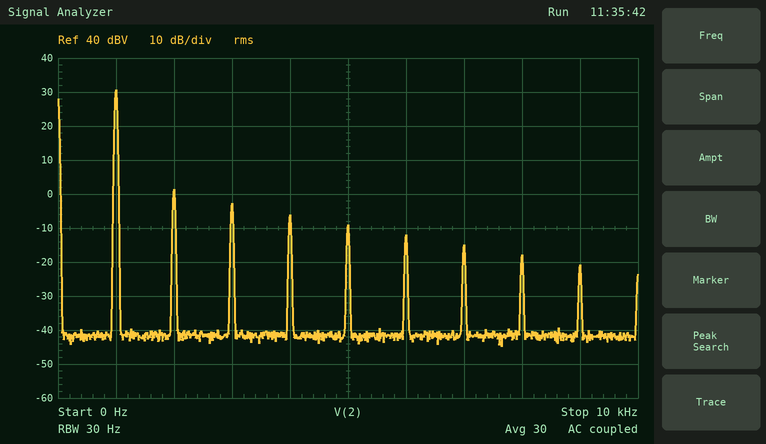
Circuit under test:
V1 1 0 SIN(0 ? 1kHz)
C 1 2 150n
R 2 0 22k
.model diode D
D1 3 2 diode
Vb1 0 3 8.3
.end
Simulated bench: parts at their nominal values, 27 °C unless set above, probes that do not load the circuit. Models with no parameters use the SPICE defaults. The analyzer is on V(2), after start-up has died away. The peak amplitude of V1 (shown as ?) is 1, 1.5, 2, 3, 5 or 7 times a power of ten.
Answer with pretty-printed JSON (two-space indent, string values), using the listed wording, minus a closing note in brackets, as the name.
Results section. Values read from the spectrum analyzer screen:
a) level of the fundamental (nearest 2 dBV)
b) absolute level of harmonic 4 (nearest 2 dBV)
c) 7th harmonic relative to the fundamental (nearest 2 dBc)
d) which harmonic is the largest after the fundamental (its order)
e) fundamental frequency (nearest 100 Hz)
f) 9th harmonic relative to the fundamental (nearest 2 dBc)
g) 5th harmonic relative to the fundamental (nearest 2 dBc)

{
  "level of the fundamental": "30 dBV",
  "absolute level of harmonic 4": "-6 dBV",
  "7th harmonic relative to the fundamental": "-46 dBc",
  "which harmonic is the largest after the fundamental": "2",
  "fundamental frequency": "1.0 kHz",
  "9th harmonic relative to the fundamental": "-52 dBc",
  "5th harmonic relative to the fundamental": "-40 dBc"
}
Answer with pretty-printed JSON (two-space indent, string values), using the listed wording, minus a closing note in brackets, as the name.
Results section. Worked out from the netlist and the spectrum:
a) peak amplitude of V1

{
  "peak amplitude of V1": "50 V"
}
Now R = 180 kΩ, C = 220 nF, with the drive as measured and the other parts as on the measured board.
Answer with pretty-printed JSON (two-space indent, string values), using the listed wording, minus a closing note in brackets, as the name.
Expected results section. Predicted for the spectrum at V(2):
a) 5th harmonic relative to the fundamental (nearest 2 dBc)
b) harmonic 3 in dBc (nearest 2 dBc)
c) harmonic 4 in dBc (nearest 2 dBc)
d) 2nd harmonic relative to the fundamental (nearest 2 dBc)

{
  "5th harmonic relative to the fundamental": "-58 dBc",
  "harmonic 3 in dBc": "-54 dBc",
  "harmonic 4 in dBc": "-56 dBc",
  "2nd harmonic relative to the fundamental": "-50 dBc"
}
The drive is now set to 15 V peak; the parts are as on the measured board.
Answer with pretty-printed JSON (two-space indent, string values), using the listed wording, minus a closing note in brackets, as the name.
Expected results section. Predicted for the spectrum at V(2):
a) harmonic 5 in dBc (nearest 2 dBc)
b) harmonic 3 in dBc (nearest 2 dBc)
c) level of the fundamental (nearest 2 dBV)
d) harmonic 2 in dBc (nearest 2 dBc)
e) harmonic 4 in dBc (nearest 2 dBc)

{
  "harmonic 5 in dBc": "-44 dBc",
  "harmonic 3 in dBc": "-40 dBc",
  "level of the fundamental": "20 dBV",
  "harmonic 2 in dBc": "-36 dBc",
  "harmonic 4 in dBc": "-42 dBc"
}
